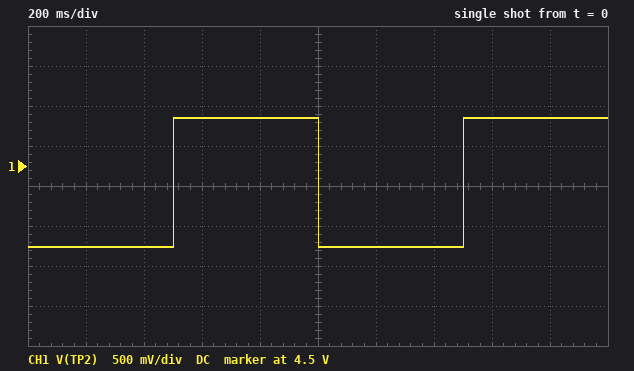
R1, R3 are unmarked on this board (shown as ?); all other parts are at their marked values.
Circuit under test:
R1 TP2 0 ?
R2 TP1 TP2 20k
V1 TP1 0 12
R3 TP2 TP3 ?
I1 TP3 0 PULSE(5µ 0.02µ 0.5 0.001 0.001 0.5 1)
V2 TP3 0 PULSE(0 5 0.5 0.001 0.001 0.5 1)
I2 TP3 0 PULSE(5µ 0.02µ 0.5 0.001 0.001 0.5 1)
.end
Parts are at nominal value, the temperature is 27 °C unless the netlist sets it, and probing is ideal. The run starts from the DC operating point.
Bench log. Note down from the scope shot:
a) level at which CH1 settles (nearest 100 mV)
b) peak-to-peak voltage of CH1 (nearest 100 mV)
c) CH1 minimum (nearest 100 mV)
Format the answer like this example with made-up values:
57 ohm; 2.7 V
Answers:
5.1 V; 1.6 V; 3.5 V
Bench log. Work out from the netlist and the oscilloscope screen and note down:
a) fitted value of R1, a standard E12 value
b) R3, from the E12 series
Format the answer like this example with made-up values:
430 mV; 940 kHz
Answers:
15 kΩ; 18 kΩ
